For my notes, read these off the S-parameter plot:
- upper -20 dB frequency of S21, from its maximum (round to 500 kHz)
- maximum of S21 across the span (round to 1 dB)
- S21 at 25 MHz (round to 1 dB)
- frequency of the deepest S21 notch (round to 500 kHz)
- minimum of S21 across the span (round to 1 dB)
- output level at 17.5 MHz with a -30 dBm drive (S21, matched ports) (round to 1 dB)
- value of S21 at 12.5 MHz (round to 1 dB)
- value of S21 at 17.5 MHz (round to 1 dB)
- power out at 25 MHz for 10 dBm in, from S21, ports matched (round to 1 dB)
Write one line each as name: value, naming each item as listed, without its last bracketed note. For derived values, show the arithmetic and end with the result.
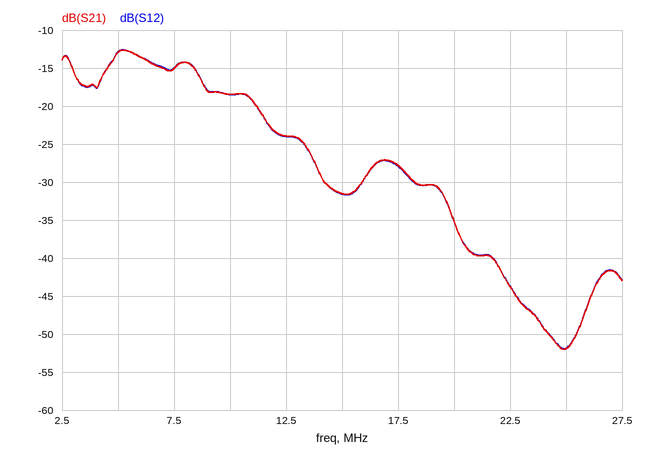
upper -20 dB frequency of S21, from its maximum: 19.5 MHz
maximum of S21 across the span: -13 dB
S21 at 25 MHz: -52 dB
frequency of the deepest S21 notch: 25.0 MHz
minimum of S21 across the span: -52 dB
output level at 17.5 MHz with a -30 dBm drive (S21, matched ports): -30 dBm + (-28 dB) = -58 dBm
value of S21 at 12.5 MHz: -24 dB
value of S21 at 17.5 MHz: -28 dB
power out at 25 MHz for 10 dBm in, from S21, ports matched: 10 dBm + (-52 dB) = -42 dBm
